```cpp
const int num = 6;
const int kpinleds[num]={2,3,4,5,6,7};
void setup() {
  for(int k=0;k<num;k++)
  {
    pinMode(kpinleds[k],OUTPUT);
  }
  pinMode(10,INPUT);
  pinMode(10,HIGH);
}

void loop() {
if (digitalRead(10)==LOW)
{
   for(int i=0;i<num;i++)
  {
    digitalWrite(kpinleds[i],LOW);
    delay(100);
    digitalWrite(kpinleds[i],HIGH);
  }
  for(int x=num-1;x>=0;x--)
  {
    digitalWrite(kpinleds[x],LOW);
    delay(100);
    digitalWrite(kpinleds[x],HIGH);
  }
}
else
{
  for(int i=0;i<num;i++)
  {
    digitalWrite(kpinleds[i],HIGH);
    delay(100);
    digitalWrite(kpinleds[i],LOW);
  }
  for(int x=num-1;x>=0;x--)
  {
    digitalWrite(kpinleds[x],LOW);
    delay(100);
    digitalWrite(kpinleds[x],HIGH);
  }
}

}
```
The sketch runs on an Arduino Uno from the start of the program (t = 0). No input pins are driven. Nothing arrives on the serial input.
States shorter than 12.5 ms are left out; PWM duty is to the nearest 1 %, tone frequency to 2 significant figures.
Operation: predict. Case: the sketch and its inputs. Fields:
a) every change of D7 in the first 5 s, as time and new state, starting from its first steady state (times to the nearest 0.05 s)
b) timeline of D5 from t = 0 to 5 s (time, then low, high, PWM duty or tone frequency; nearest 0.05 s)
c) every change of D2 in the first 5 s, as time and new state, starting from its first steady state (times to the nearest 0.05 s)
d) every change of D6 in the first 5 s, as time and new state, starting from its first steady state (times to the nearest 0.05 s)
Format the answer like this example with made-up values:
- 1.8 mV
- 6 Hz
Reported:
- 0 s low; 0.7 s high; 1.7 s low; 1.9 s high; 2.9 s low; 3.1 s high; 4.1 s low; 4.3 s high
- 0 s low; 0.4 s high; 0.8 s low; 0.9 s high; 1.5 s low; 1.6 s high; 2 s low; 2.1 s high; 2.7 s low; 2.8 s high; 3.2 s low; 3.3 s high; 3.9 s low; 4 s high; 4.4 s low; 4.5 s high
- 0 s low; 0.1 s high; 1.1 s low; 1.3 s high; 2.3 s low; 2.5 s high; 3.5 s low; 3.7 s high; 4.7 s low; 4.9 s high
- 0 s low; 0.5 s high; 0.7 s low; 0.8 s high; 1.6 s low; 1.7 s high; 1.9 s low; 2 s high; 2.8 s low; 2.9 s high; 3.1 s low; 3.2 s high; 4 s low; 4.1 s high; 4.3 s low; 4.4 s high
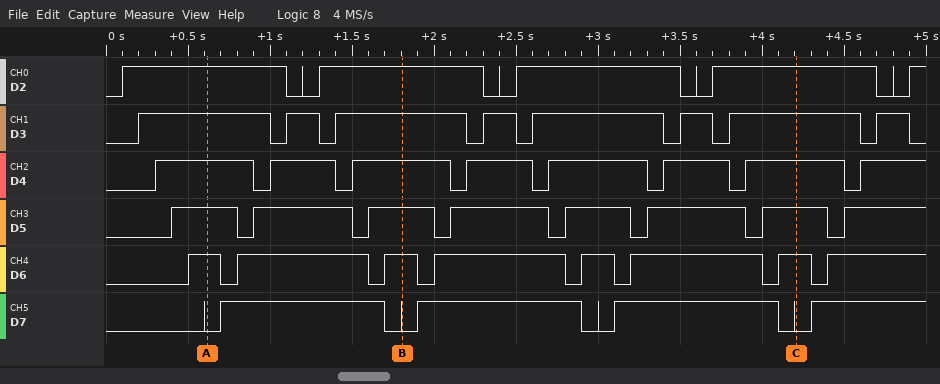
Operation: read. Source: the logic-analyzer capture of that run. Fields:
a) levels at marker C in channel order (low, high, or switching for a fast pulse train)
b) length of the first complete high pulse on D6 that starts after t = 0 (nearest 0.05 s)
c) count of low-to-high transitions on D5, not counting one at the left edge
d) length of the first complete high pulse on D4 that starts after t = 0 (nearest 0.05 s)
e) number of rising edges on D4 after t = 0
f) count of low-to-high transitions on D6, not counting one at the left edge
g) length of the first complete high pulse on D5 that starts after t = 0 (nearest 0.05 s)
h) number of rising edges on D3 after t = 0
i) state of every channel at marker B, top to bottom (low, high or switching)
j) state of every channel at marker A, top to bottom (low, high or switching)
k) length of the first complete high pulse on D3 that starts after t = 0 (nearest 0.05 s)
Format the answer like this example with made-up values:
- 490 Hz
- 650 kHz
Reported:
- D2 high, D3 high, D4 high, D5 high, D6 high, D7 low
- 0.20 s
- 8
- 0.60 s
- 8
- 8
- 0.40 s
- 8
- D2 high, D3 high, D4 high, D5 high, D6 high, D7 low
- D2 high, D3 high, D4 high, D5 high, D6 high, D7 low
- 0.80 s
